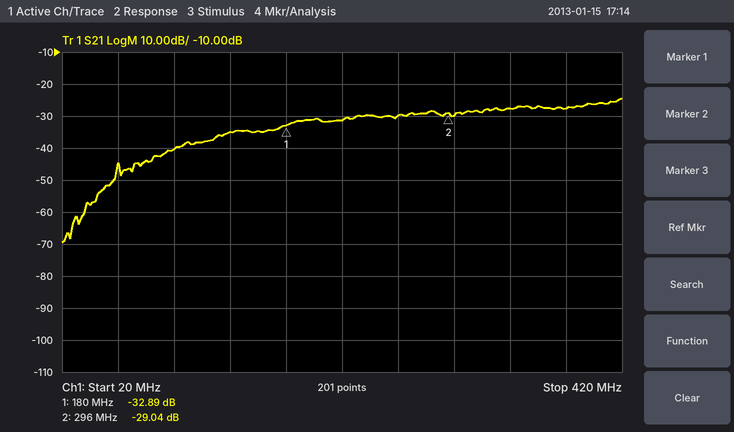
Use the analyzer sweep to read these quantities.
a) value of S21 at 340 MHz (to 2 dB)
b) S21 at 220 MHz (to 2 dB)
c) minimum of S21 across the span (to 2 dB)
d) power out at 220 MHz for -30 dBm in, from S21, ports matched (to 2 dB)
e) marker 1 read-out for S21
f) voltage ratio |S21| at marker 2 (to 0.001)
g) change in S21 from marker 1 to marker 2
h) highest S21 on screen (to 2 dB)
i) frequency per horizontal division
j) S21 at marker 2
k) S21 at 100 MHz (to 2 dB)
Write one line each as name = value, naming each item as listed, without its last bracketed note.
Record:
value of S21 at 340 MHz = -28 dB
S21 at 220 MHz = -32 dB
minimum of S21 across the span = -70 dB
power out at 220 MHz for -30 dBm in, from S21, ports matched = -62 dBm
marker 1 read-out for S21 = -32.89 dB
voltage ratio |S21| at marker 2 = 0.035
change in S21 from marker 1 to marker 2 = 3.85 dB
highest S21 on screen = -24 dB
frequency per horizontal division = 40 MHz
S21 at marker 2 = -29.04 dB
S21 at 100 MHz = -40 dB
